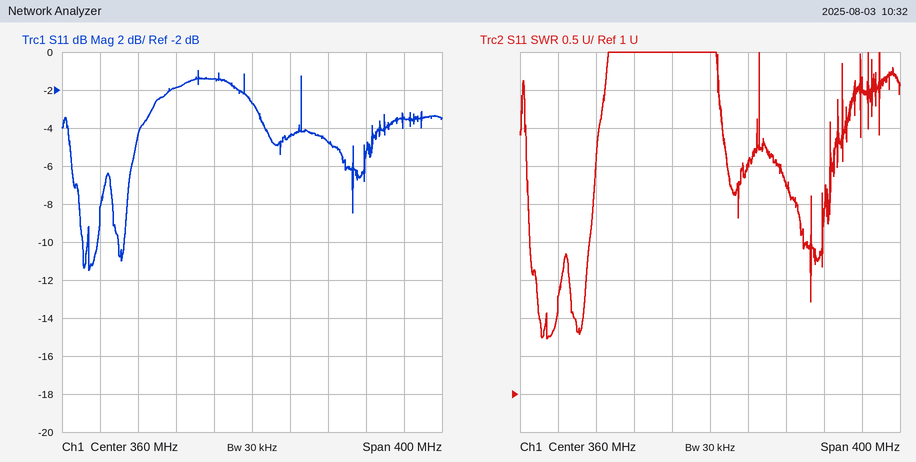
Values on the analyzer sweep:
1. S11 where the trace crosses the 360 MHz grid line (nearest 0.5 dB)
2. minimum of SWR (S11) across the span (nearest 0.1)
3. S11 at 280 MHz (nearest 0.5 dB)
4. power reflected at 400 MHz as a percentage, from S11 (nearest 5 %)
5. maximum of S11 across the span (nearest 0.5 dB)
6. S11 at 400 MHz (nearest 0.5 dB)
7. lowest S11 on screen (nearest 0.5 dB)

-2.5 dB
1.7
-2.0 dB
35 %
-1.0 dB
-4.5 dB
-11.5 dB
